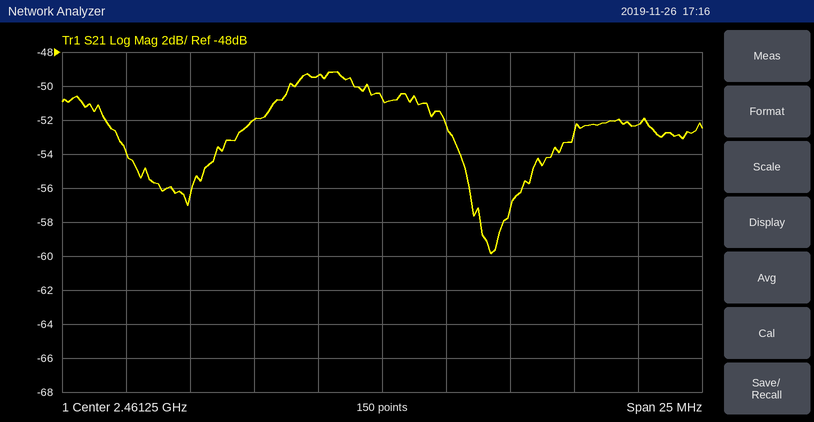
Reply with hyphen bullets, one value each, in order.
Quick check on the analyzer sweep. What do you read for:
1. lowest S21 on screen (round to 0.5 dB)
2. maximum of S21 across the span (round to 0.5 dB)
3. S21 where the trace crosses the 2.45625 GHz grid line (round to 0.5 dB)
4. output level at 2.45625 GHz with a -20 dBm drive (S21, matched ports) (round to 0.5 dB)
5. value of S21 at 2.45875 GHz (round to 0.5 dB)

- -60.0 dB
- -49.0 dB
- -52.0 dB
- -72.0 dBm
- -49.5 dB
